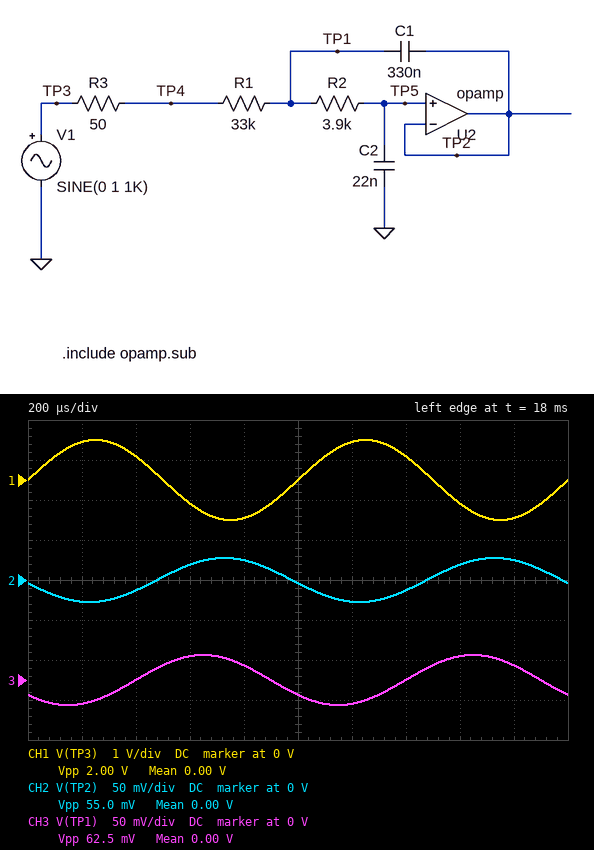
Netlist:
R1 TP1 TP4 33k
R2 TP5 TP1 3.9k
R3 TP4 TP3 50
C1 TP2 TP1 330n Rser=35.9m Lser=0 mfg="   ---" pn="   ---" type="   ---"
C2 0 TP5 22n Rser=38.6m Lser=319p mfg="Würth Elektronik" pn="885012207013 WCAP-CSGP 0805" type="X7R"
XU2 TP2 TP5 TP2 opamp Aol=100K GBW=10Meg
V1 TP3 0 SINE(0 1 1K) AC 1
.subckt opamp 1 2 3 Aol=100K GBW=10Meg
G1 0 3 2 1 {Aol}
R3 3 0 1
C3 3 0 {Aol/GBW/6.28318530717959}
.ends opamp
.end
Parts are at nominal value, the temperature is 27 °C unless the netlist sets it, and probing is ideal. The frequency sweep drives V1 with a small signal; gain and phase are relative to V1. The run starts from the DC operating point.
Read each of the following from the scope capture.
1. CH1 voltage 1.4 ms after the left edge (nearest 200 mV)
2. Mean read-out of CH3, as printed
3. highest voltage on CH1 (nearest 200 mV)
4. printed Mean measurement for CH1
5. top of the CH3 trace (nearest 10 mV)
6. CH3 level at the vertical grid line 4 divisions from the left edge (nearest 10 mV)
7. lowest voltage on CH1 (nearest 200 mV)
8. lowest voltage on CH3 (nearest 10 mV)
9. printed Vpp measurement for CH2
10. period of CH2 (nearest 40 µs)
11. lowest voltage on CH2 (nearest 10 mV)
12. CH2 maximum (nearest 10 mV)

600 mV
0.00 V
1.0 V
0.00 V
30 mV
20 mV
-1.0 V
-30 mV
55.0 mV
1.00 ms
-30 mV
30 mV
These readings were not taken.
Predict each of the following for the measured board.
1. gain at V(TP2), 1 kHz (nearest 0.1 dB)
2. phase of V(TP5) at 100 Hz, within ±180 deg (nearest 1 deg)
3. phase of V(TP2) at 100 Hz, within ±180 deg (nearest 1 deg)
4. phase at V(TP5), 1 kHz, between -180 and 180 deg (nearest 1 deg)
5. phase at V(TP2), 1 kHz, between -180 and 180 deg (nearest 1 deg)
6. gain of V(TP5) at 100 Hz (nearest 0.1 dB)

-31.2 dB
-39 deg
-39 deg
-172 deg
-172 deg
1.8 dB
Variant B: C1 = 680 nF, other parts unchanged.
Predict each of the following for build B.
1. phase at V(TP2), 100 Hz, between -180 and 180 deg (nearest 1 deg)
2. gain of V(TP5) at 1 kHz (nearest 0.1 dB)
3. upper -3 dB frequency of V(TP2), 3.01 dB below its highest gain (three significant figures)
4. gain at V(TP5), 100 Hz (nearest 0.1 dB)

-65 deg
-37.5 dB
135 Hz
5.0 dB
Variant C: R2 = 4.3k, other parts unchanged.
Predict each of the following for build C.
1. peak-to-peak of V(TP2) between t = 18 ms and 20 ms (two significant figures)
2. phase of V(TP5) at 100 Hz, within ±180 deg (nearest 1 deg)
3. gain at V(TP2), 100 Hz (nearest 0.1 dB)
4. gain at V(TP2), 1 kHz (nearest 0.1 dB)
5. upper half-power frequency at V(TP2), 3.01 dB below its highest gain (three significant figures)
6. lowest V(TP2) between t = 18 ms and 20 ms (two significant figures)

50 mV
-41 deg
2.1 dB
-32.1 dB
186 Hz
-25 mV
